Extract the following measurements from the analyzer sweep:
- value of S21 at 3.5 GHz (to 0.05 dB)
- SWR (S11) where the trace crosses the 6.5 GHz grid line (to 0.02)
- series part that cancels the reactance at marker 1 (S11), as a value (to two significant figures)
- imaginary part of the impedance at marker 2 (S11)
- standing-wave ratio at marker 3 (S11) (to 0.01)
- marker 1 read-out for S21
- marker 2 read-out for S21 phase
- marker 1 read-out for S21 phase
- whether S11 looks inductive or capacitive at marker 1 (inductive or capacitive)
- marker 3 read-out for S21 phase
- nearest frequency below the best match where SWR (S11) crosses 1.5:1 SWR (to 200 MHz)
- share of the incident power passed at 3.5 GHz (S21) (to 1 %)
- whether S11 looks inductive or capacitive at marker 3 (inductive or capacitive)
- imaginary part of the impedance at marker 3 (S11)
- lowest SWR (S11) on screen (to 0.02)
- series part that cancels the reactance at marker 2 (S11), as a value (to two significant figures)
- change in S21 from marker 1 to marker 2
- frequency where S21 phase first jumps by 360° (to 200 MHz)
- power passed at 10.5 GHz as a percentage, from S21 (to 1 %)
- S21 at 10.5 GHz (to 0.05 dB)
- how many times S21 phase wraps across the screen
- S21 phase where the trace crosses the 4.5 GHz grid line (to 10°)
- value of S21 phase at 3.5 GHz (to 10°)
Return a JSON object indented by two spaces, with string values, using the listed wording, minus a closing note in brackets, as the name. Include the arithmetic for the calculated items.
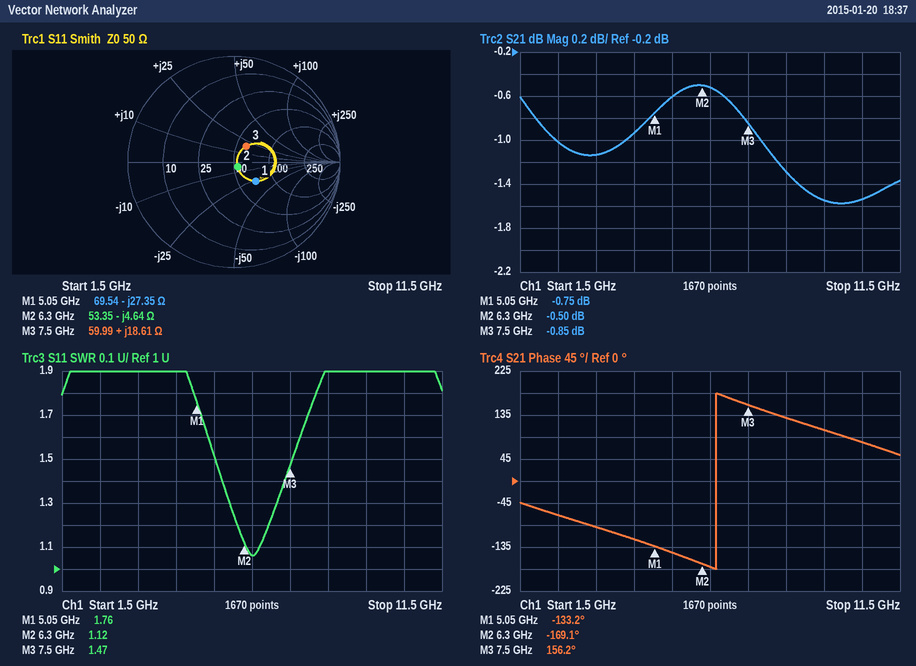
{
  "value of S21 at 3.5 GHz": "-1.15 dB",
  "SWR (S11) where the trace crosses the 6.5 GHz grid line": "1.06",
  "series part that cancels the reactance at marker 1 (S11), as a value": "L = 27.35 Ω/(2π × 5.05 GHz) ≈ 862 pH, so 860 pH to two significant figures",
  "imaginary part of the impedance at marker 2": "-4.64 Ω",
  "standing-wave ratio at marker 3 (S11)": "1.47",
  "marker 1 read-out for S21": "-0.75 dB",
  "marker 2 read-out for S21 phase": "-169.1°",
  "marker 1 read-out for S21 phase": "-133.2°",
  "whether S11 looks inductive or capacitive at marker 1": "capacitive",
  "marker 3 read-out for S21 phase": "156.2°",
  "nearest frequency below the best match where SWR (S11) crosses 1.5:1 SWR": "5.6 GHz",
  "share of the incident power passed at 3.5 GHz (S21)": "10^(-1.15/10) ≈ 77 %",
  "whether S11 looks inductive or capacitive at marker 3": "inductive",
  "imaginary part of the impedance at marker 3": "+18.61 Ω",
  "lowest SWR (S11) on screen": "1.06",
  "series part that cancels the reactance at marker 2 (S11), as a value": "L = 4.64 Ω/(2π × 6.3 GHz) ≈ 117 pH, so 120 pH to two significant figures",
  "change in S21 from marker 1 to marker 2": "-0.5 − (-0.75) = 0.25 dB",
  "frequency where S21 phase first jumps by 360°": "6.6 GHz",
  "power passed at 10.5 GHz as a percentage, from S21": "10^(-1.55/10) ≈ 70 %",
  "S21 at 10.5 GHz": "-1.55 dB",
  "how many times S21 phase wraps across the screen": "1",
  "S21 phase where the trace crosses the 4.5 GHz grid line": "-120°",
  "value of S21 phase at 3.5 GHz": "-90°"
}
